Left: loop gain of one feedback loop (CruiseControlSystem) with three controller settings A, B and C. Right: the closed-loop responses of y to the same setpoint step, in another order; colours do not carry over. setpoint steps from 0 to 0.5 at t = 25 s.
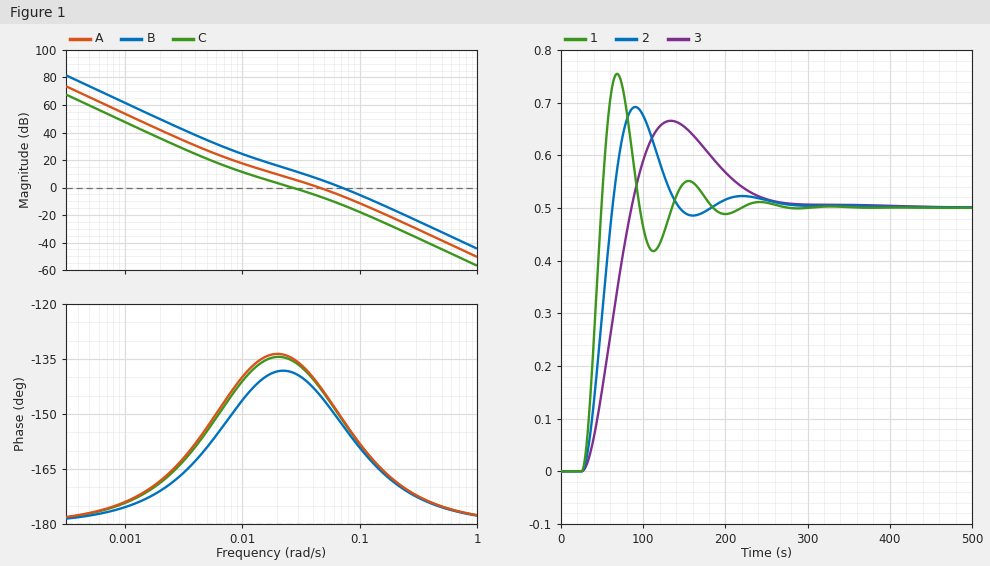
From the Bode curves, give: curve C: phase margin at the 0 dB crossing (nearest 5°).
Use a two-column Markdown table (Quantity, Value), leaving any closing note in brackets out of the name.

| Quantity | Value |
|---|---|
| curve C: phase margin at the 0 dB crossing | 45° |
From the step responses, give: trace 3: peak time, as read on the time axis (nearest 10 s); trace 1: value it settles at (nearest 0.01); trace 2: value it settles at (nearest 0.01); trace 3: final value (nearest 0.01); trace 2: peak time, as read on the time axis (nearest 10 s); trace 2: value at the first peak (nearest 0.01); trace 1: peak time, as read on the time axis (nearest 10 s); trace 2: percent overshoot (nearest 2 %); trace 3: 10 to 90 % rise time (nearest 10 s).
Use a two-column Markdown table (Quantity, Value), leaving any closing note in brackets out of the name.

| Quantity | Value |
|---|---|
| trace 3: peak time, as read on the time axis | 130 s |
| trace 1: value it settles at | 0.50 |
| trace 2: value it settles at | 0.50 |
| trace 3: final value | 0.50 |
| trace 2: peak time, as read on the time axis | 90 s |
| trace 2: value at the first peak | 0.69 |
| trace 1: peak time, as read on the time axis | 70 s |
| trace 2: percent overshoot | 38 % |
| trace 3: 10 to 90 % rise time | 40 s |
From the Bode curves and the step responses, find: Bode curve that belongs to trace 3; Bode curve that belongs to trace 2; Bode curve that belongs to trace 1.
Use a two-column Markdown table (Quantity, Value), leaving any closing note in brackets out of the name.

| Quantity | Value |
|---|---|
| Bode curve that belongs to trace 3 | C |
| Bode curve that belongs to trace 2 | A |
| Bode curve that belongs to trace 1 | B |
